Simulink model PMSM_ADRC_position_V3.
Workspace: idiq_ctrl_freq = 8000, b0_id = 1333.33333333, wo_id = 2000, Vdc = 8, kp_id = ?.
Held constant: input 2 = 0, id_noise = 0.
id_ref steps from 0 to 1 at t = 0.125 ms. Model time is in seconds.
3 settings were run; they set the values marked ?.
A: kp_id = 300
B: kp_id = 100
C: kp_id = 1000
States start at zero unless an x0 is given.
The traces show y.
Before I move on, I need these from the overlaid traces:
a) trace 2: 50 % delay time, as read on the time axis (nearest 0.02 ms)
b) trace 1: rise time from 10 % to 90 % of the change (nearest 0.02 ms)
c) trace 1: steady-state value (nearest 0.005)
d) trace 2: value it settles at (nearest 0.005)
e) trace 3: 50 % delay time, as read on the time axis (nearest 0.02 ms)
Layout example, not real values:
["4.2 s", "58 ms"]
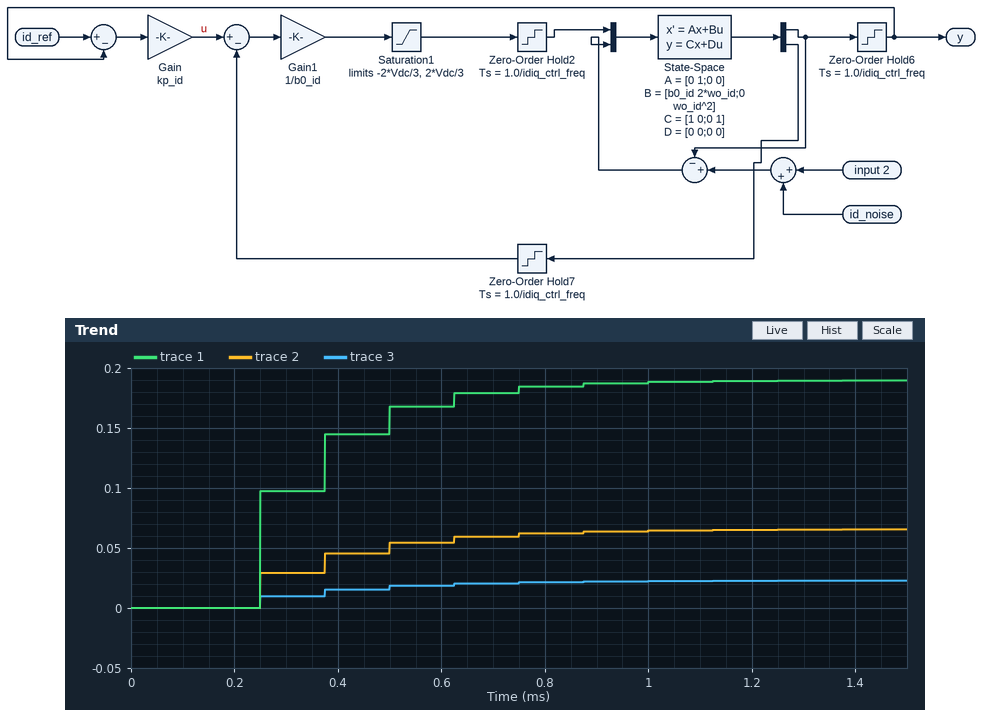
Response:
["0.38 ms", "0.38 ms", "0.190", "0.065", "0.38 ms"]
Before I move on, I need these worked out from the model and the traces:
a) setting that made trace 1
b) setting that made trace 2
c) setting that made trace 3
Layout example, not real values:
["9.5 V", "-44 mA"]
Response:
["C", "A", "B"]
